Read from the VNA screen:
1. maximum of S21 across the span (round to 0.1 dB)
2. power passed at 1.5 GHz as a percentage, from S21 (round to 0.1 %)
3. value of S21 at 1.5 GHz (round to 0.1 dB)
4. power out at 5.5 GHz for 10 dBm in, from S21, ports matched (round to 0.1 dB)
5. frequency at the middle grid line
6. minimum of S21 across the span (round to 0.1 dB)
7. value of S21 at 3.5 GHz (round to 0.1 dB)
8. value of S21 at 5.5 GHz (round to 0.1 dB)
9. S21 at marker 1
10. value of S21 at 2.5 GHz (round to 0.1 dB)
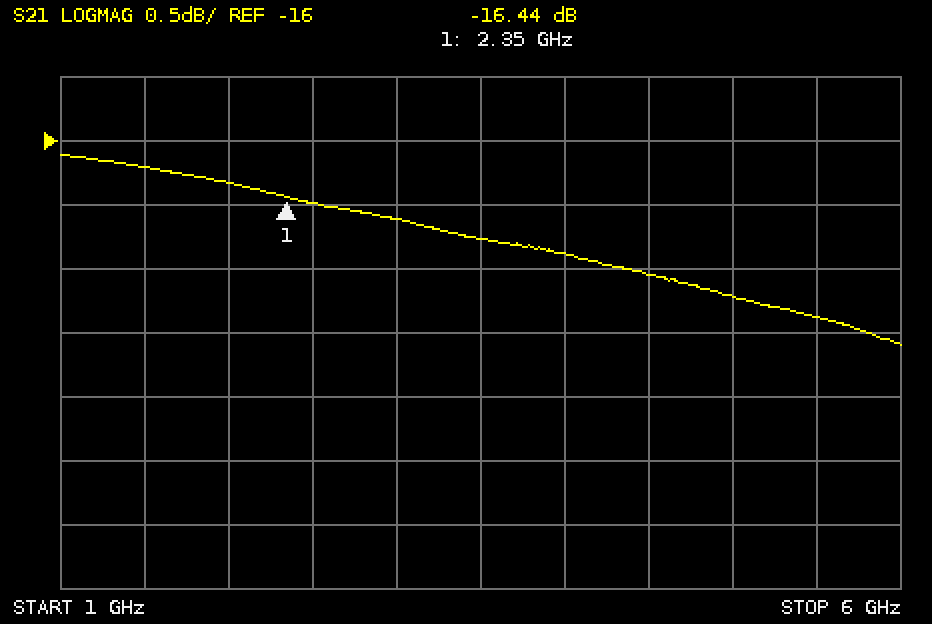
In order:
-16.1 dB
2.4 %
-16.2 dB
-7.4 dBm
3.5 GHz
-17.6 dB
-16.8 dB
-17.4 dB
-16.44 dB
-16.5 dB
